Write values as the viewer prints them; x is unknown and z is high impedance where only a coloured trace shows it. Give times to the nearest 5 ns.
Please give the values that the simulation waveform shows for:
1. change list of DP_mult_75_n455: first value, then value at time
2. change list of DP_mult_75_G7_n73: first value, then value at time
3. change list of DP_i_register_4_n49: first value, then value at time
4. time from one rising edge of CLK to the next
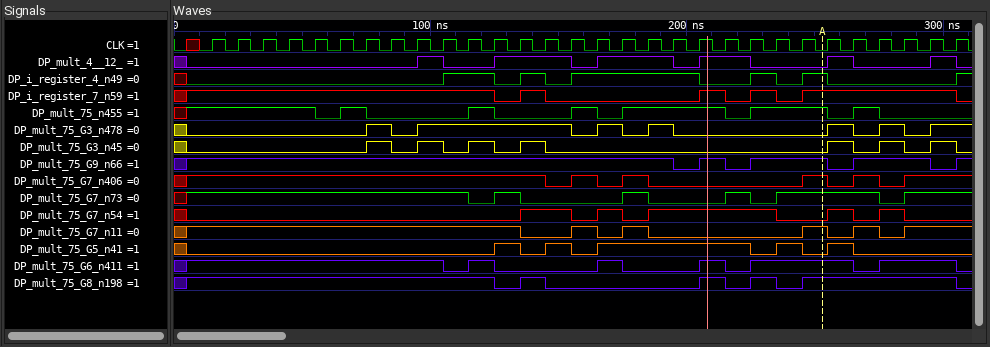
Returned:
x, 1 at 5 ns, 0 at 55 ns, 1 at 65 ns, 0 at 75 ns, 1 at 115 ns, 0 at 125 ns, 1 at 155 ns, 0 at 165 ns, 1 at 175 ns, 0 at 215 ns, 1 at 225 ns, 0 at 255 ns, 1 at 265 ns, 0 at 275 ns
x, 1 at 5 ns, 0 at 115 ns, 1 at 125 ns, 0 at 135 ns, 1 at 175 ns, 0 at 185 ns, 1 at 215 ns, 0 at 225 ns, 1 at 235 ns, 0 at 275 ns, 1 at 285 ns
x, 0 at 5 ns, 1 at 105 ns, 0 at 125 ns, 1 at 135 ns, 0 at 145 ns, 1 at 155 ns, 0 at 205 ns, 1 at 225 ns, 0 at 235 ns, 1 at 245 ns, 0 at 255 ns, 1 at 305 ns
10 ns
